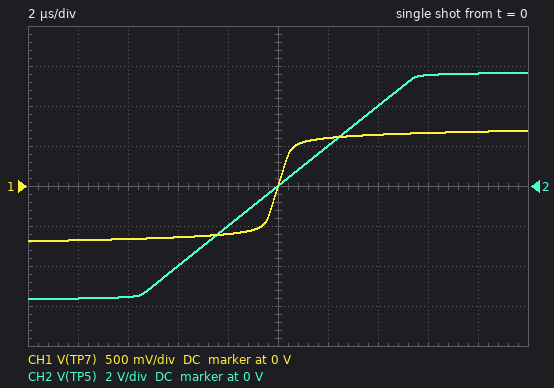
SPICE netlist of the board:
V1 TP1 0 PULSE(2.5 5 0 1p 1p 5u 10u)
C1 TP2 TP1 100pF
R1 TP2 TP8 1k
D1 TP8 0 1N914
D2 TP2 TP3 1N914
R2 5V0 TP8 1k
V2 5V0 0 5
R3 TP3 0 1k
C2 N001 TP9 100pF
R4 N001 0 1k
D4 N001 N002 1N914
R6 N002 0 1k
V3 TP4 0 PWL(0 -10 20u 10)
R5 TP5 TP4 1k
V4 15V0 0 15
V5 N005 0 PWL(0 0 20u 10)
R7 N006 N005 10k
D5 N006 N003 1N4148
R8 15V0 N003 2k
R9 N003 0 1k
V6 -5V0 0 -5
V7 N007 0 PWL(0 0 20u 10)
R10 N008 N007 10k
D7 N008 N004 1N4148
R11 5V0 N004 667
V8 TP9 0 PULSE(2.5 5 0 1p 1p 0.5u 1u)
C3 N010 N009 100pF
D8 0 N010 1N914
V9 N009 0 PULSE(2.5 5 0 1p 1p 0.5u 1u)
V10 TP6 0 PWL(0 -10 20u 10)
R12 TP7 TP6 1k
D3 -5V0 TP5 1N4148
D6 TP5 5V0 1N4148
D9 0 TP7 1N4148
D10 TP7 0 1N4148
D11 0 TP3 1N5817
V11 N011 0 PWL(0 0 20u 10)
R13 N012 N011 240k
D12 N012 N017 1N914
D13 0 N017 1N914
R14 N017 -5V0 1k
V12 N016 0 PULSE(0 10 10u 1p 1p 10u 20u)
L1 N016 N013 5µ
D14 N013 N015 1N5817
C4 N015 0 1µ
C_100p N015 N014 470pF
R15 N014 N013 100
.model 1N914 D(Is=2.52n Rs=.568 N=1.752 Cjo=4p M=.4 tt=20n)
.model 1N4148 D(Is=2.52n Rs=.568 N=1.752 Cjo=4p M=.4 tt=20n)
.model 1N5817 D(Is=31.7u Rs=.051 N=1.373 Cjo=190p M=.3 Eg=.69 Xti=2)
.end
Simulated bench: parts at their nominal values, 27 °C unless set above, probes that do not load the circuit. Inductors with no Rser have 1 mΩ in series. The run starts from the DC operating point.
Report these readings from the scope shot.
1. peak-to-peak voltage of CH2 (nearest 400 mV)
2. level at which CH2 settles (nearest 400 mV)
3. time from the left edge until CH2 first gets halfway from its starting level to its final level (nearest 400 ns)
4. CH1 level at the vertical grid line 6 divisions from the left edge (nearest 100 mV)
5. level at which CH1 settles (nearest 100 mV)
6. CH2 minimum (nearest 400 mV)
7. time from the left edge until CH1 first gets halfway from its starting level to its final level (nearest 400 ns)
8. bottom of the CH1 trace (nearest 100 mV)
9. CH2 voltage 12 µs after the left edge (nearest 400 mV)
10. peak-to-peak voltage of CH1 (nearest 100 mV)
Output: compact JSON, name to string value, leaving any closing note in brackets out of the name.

{"peak-to-peak voltage of CH2": "11.2 V", "level at which CH2 settles": "5.6 V", "time from the left edge until CH2 first gets halfway from its starting level to its final level": "10.0 µs", "CH1 level at the vertical grid line 6 divisions from the left edge": "600 mV", "level at which CH1 settles": "700 mV", "CH2 minimum": "-5.6 V", "time from the left edge until CH1 first gets halfway from its starting level to its final level": "10.0 µs", "bottom of the CH1 trace": "-700 mV", "CH2 voltage 12 µs after the left edge": "2.0 V", "peak-to-peak voltage of CH1": "1.4 V"}
